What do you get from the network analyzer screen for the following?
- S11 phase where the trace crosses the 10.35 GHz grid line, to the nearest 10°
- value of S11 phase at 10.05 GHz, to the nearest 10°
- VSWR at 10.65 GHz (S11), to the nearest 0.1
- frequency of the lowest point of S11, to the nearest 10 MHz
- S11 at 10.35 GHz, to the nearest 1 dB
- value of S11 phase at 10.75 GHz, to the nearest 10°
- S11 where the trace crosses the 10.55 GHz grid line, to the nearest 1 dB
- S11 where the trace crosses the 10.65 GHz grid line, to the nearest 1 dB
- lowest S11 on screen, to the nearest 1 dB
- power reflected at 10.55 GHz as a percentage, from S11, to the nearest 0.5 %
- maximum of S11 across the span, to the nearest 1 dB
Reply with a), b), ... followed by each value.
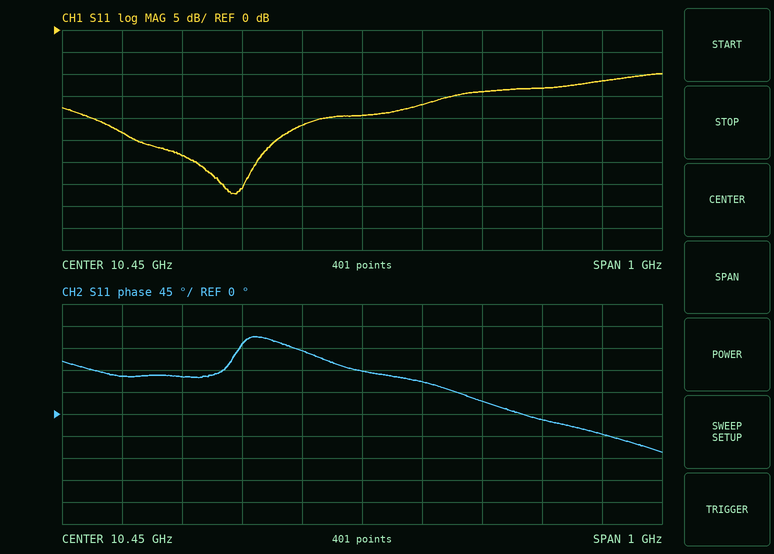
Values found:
a) 130°
b) 80°
c) 1.5
d) 10.23 GHz
e) -22 dB
f) -10°
g) -17 dB
h) -14 dB
i) -37 dB
j) 2.0 %
k) -10 dB
